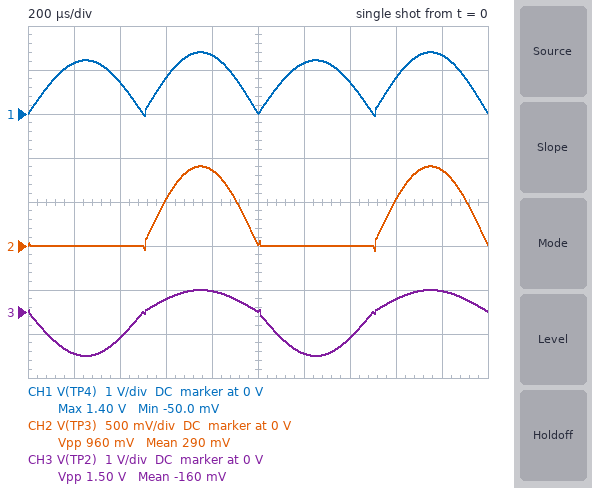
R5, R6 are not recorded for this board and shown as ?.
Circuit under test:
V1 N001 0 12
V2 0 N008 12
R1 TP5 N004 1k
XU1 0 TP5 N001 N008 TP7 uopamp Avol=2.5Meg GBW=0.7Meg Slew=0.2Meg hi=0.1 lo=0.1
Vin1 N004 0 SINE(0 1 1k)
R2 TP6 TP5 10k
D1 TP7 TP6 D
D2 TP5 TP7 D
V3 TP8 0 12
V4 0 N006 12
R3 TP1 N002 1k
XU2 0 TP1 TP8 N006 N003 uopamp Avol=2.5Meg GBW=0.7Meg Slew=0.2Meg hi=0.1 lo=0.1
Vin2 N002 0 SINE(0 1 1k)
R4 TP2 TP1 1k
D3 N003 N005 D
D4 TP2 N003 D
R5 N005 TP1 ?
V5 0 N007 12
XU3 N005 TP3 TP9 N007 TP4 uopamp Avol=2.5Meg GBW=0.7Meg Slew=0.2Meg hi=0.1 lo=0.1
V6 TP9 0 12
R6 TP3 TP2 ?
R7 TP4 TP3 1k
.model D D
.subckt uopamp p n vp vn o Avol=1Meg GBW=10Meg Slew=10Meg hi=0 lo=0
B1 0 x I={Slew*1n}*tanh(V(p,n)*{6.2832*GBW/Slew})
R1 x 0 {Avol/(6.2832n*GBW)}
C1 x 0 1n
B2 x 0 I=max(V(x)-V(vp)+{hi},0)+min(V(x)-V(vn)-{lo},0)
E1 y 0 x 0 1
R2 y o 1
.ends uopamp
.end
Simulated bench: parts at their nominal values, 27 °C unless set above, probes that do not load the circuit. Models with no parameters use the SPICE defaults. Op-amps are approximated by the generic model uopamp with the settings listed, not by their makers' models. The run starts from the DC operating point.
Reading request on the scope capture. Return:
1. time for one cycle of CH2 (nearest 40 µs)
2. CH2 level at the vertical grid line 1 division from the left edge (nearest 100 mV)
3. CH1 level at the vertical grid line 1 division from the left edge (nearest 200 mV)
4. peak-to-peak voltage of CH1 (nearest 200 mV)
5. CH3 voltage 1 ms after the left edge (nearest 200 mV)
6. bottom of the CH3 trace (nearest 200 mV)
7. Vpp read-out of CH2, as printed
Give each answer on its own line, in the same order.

1.00 ms
0 V
1.2 V
1.4 V
0 V
-1.0 V
960 mV
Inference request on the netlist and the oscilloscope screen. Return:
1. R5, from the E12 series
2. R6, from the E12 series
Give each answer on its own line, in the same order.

1.8 kΩ
820 Ω
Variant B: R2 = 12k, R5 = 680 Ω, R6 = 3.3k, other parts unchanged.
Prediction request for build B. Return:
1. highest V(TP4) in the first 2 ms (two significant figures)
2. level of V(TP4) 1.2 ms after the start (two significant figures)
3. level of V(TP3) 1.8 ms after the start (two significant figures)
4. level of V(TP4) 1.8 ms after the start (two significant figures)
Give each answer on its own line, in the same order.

720 mV
290 mV
560 mV
690 mV
